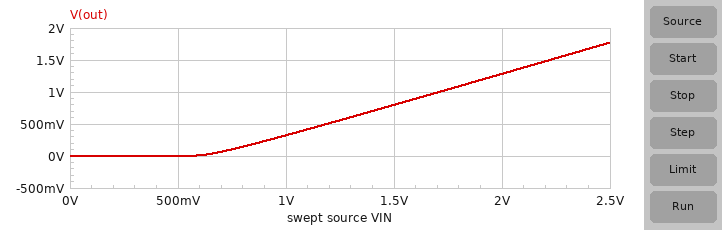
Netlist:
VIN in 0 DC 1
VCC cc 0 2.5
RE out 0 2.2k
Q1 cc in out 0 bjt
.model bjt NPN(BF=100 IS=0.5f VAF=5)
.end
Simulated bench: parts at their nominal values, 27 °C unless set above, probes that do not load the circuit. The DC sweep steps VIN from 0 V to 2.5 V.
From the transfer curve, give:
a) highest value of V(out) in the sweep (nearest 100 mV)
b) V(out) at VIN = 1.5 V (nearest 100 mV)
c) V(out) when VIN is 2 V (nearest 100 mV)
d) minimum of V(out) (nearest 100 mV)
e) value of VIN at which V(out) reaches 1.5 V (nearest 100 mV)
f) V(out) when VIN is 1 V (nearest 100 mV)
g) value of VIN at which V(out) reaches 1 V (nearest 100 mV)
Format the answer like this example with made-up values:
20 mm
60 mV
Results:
1.8 V
800 mV
1.3 V
0 V
2.2 V
300 mV
1.7 V
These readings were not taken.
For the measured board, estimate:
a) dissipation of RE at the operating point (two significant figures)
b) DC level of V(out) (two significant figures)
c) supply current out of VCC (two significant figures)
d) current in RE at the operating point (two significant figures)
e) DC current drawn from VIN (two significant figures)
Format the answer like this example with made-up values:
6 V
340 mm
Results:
48 µW
320 mV
150 µA
150 µA
1.1 µA
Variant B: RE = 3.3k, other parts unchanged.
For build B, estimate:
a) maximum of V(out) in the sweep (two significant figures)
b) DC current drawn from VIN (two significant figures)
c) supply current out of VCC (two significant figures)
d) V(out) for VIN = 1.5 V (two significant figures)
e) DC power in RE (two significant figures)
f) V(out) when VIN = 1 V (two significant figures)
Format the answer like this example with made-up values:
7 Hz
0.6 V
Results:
1.8 V
770 nA
100 µA
810 mV
34 µW
330 mV
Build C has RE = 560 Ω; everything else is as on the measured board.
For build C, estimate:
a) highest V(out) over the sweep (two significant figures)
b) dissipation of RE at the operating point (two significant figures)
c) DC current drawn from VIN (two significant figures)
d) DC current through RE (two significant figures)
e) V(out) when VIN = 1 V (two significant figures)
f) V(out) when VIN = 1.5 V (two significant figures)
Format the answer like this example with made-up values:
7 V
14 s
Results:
1.7 V
150 µW
4.0 µA
520 µA
290 mV
760 mV
